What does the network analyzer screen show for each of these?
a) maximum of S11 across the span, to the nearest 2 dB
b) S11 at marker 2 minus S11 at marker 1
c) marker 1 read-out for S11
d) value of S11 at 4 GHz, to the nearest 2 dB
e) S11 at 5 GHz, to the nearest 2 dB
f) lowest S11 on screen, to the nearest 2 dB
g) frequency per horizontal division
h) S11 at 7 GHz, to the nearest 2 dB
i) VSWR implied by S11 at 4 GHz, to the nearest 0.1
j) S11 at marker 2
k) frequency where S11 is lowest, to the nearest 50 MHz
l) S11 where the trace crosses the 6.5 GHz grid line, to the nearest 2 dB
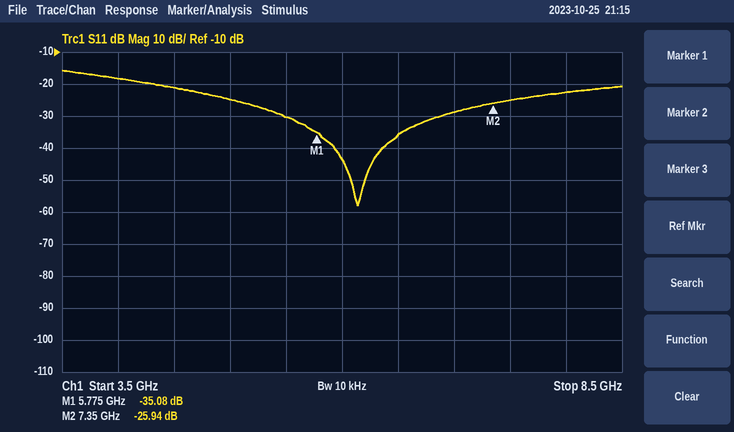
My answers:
-16 dB
9.14 dB
-35.08 dB
-18 dB
-24 dB
-58 dB
500 MHz
-28 dB
1.3
-25.94 dB
6.15 GHz
-36 dB
